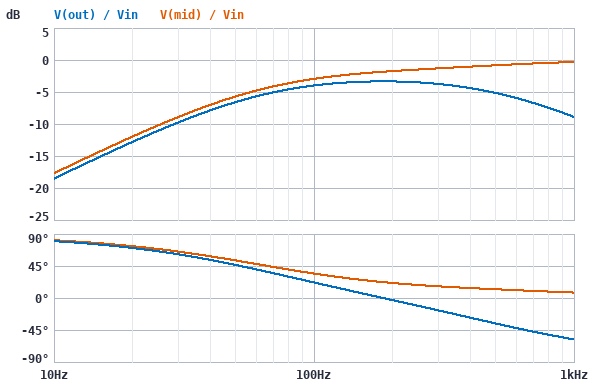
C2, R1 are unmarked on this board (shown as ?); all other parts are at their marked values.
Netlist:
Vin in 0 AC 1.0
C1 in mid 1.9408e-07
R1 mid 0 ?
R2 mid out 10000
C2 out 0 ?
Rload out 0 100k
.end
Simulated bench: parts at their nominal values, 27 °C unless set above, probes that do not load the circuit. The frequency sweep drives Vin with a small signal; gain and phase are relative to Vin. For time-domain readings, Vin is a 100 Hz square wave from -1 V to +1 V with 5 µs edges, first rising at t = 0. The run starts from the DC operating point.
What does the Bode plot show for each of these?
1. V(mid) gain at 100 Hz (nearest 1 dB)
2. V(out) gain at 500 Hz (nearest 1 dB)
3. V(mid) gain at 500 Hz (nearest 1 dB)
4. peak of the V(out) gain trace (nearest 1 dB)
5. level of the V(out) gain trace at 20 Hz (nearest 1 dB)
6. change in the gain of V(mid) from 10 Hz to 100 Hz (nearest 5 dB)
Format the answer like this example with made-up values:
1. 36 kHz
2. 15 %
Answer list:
1. -3 dB
2. -5 dB
3. -1 dB
4. -3 dB
5. -13 dB
6. 15 dB
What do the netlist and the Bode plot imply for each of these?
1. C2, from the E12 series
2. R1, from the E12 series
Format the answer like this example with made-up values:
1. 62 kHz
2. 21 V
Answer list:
1. 39 nF
2. 12 kΩ
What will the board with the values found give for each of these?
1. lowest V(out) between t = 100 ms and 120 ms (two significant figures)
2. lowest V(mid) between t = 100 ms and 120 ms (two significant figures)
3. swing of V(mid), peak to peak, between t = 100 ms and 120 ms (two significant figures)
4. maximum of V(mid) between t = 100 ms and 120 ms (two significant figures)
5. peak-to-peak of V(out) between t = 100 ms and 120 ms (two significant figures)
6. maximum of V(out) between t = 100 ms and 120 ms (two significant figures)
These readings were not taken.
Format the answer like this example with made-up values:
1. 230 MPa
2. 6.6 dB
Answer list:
1. -990 mV
2. -1.8 V
3. 3.6 V
4. 1.8 V
5. 2.0 V
6. 990 mV
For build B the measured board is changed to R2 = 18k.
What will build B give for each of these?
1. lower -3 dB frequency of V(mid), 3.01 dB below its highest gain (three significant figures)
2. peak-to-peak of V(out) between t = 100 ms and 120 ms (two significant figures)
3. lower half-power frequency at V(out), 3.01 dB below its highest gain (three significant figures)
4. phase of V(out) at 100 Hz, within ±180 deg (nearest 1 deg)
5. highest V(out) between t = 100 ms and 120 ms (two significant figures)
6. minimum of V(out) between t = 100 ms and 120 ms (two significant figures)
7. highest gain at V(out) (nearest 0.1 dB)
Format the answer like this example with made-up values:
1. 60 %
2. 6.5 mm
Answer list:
1. 93.3 Hz
2. 1.6 V
3. 47.0 Hz
4. 15 deg
5. 810 mV
6. -810 mV
7. -4.5 dB
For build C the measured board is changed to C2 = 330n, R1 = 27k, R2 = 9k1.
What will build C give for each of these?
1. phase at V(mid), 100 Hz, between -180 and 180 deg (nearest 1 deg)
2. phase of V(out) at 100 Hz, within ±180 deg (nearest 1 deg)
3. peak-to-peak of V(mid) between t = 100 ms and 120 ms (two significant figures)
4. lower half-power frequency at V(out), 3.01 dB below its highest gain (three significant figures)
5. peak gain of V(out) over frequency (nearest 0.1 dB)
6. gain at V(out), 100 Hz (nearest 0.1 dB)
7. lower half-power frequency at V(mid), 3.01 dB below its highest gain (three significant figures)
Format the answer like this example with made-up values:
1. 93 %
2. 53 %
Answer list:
1. 36 deg
2. -24 deg
3. 3.5 V
4. 11.5 Hz
5. -10.5 dB
6. -11.3 dB
7. 145 Hz
